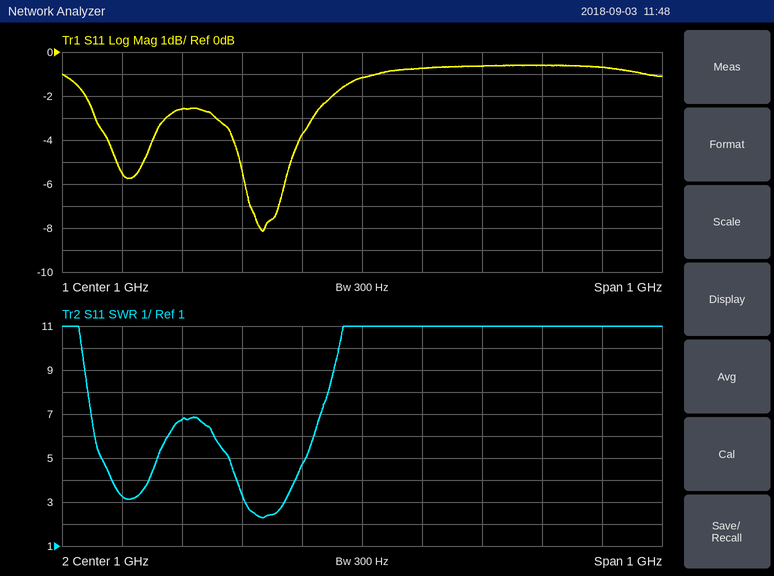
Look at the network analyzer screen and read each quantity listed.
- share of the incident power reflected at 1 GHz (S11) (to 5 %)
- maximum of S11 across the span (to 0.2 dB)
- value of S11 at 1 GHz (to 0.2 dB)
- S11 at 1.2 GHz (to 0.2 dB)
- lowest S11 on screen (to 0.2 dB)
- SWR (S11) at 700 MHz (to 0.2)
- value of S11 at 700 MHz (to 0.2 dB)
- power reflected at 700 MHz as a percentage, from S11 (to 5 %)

75 %
-0.6 dB
-1.2 dB
-0.6 dB
-8.2 dB
6.8
-2.6 dB
55 %
